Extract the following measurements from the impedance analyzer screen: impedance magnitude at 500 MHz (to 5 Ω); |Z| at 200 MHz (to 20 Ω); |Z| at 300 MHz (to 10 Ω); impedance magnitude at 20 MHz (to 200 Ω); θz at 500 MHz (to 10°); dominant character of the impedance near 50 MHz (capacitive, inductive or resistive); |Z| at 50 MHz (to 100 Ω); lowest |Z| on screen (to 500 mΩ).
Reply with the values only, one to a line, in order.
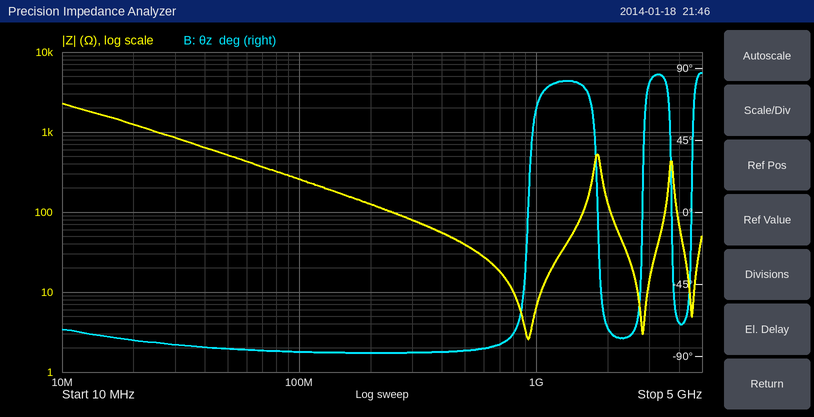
40 Ω
120 Ω
80 Ω
1.2 kΩ
-90°
capacitive
500 Ω
2.5 Ω
